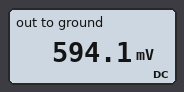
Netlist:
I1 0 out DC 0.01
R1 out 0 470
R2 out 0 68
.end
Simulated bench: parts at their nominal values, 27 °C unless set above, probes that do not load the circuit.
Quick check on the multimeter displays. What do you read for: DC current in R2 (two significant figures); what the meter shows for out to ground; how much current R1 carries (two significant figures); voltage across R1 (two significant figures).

8.7 mA
594.1 mV
1.3 mA
590 mV
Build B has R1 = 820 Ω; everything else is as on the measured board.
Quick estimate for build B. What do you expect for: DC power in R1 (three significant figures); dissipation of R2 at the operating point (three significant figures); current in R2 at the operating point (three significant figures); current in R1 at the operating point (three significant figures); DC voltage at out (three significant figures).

481 µW
5.80 mW
9.23 mA
766 µA
628 mV
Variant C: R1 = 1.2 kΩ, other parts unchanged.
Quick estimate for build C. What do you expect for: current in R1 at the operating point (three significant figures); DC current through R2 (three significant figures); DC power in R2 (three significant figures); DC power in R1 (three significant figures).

536 µA
9.46 mA
6.09 mW
345 µW
